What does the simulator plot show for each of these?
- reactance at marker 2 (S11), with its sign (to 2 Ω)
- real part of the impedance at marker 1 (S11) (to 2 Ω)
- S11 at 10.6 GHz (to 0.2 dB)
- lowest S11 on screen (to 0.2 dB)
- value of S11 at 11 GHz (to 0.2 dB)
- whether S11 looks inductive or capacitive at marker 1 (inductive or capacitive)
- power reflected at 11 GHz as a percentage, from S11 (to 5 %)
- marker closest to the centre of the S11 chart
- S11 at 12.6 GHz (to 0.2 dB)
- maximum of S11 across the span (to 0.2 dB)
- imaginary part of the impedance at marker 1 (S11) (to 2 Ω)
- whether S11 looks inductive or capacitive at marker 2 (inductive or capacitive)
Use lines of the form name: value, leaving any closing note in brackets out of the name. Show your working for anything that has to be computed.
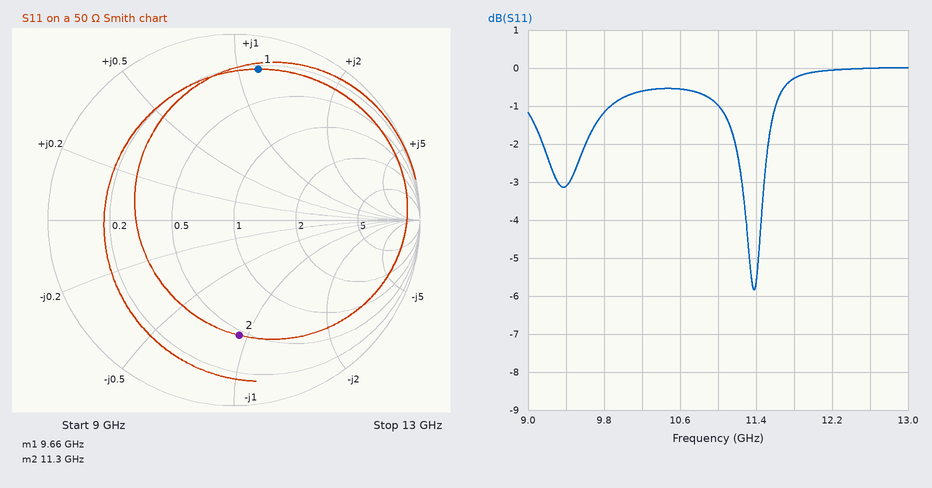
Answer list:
reactance at marker 2 (S11), with its sign: -46 Ω
real part of the impedance at marker 1 (S11): 12 Ω
S11 at 10.6 GHz: -0.6 dB
lowest S11 on screen: -5.8 dB
value of S11 at 11 GHz: -1.0 dB
whether S11 looks inductive or capacitive at marker 1: inductive
power reflected at 11 GHz as a percentage, from S11: 10^(-1/10) ≈ 79.4 %, so 80 % to the nearest 5 %
marker closest to the centre of the S11 chart: marker 2
S11 at 12.6 GHz: 0.0 dB
maximum of S11 across the span: 0.0 dB
imaginary part of the impedance at marker 1 (S11): +58 Ω
whether S11 looks inductive or capacitive at marker 2: capacitive
